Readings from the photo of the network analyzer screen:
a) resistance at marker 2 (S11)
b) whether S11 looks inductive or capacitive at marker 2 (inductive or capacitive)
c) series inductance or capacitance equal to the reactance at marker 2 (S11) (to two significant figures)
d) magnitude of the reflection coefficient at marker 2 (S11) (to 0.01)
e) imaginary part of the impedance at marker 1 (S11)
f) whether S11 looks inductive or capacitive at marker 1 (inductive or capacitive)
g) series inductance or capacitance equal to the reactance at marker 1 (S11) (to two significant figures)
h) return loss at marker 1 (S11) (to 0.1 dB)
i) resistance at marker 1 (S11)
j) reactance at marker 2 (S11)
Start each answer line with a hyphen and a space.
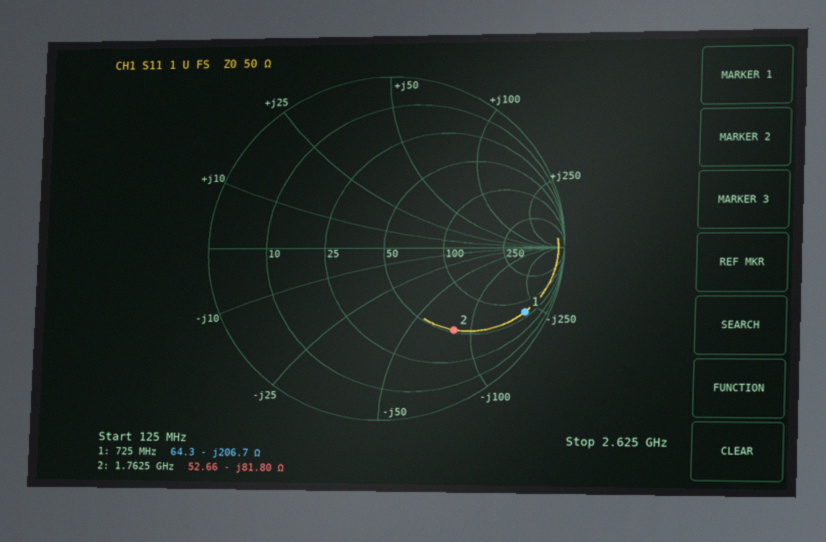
- 52.66 Ω
- capacitive
- 1.1 pF
- 0.62
- -206.7 Ω
- capacitive
- 1.1 pF
- 1.1 dB
- 64.3 Ω
- -81.80 Ω
